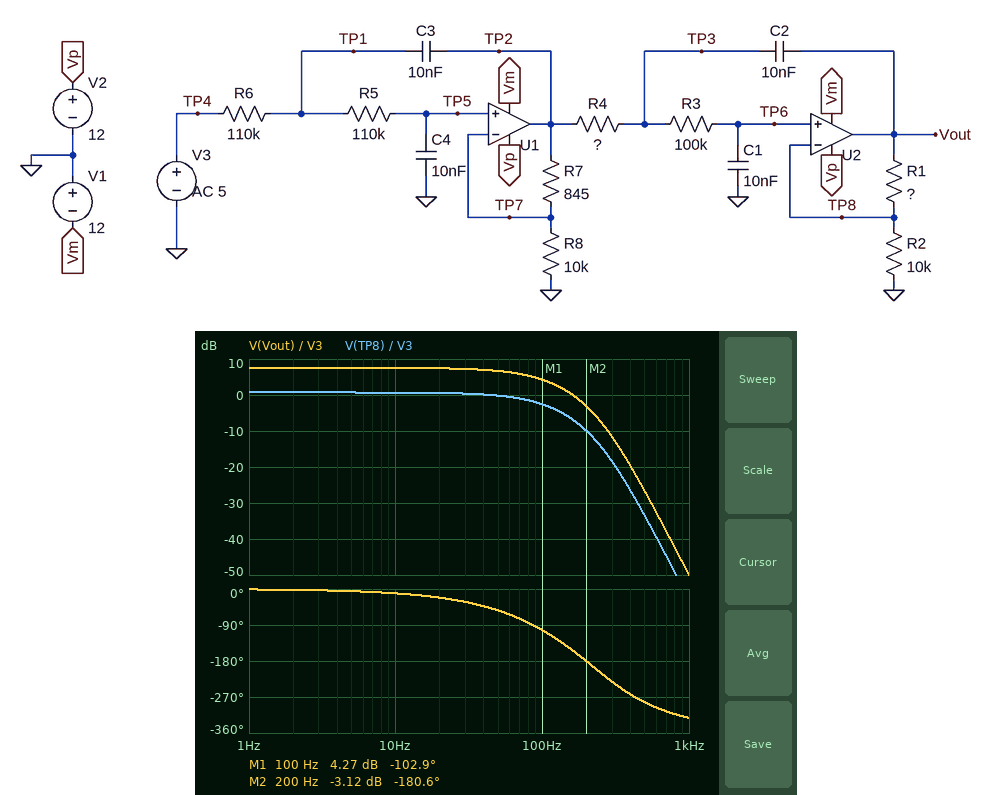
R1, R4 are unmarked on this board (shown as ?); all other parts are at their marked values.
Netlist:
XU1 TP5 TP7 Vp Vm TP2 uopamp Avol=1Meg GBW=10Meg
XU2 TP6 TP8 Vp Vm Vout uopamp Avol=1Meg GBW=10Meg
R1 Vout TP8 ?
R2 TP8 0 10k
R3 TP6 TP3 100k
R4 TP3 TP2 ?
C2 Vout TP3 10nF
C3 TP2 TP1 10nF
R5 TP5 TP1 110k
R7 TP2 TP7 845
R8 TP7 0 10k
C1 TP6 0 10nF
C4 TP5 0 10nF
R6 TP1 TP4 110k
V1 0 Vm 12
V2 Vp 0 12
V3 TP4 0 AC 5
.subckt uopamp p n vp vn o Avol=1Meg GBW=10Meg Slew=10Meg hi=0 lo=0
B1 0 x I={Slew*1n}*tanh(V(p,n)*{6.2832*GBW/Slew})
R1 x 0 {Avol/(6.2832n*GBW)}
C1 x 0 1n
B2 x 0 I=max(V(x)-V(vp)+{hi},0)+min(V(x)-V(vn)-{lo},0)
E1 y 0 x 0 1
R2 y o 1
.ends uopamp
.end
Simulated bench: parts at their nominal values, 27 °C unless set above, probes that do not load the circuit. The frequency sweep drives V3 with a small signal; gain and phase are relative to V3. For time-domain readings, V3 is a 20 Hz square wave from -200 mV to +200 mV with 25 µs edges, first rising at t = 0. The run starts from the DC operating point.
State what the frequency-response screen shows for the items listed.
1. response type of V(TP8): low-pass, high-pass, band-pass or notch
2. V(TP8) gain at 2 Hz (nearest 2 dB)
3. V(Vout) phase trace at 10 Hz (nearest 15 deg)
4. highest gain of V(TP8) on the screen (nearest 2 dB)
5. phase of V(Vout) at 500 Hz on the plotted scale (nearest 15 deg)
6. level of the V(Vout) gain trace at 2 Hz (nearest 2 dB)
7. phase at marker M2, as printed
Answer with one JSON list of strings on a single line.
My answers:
["low-pass", "0 dB", "-15 deg", "0 dB", "-285 deg", "8 dB", "-180.6 deg"]
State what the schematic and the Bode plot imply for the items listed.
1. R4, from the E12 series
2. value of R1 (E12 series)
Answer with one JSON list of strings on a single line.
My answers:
["39 kΩ", "12 kΩ"]
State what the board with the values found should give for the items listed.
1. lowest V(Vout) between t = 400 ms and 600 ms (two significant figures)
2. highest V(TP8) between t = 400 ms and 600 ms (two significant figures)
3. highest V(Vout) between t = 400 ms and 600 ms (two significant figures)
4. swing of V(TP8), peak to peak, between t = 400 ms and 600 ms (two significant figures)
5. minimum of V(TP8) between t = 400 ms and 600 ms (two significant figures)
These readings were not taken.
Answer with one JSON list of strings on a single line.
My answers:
["-480 mV", "220 mV", "480 mV", "430 mV", "-220 mV"]
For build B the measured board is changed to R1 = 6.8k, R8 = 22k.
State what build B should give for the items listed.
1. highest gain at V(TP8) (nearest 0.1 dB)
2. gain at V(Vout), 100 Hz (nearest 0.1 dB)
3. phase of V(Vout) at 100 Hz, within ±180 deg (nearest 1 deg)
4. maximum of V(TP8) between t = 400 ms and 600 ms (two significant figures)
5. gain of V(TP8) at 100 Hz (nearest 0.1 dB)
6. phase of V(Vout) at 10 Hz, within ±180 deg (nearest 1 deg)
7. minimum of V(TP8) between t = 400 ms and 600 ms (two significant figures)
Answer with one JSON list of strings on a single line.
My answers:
["0.3 dB", "0.7 dB", "-109 deg", "210 mV", "-3.8 dB", "-12 deg", "-210 mV"]
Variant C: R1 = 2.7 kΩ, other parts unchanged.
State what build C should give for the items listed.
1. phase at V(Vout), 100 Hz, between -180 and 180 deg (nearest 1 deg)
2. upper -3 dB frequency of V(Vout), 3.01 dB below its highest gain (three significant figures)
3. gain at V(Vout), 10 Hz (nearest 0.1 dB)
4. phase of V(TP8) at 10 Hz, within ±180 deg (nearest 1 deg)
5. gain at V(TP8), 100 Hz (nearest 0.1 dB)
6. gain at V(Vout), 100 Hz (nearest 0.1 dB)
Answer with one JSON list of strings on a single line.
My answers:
["-112 deg", "80.9 Hz", "2.7 dB", "-12 deg", "-3.7 dB", "-1.6 dB"]
